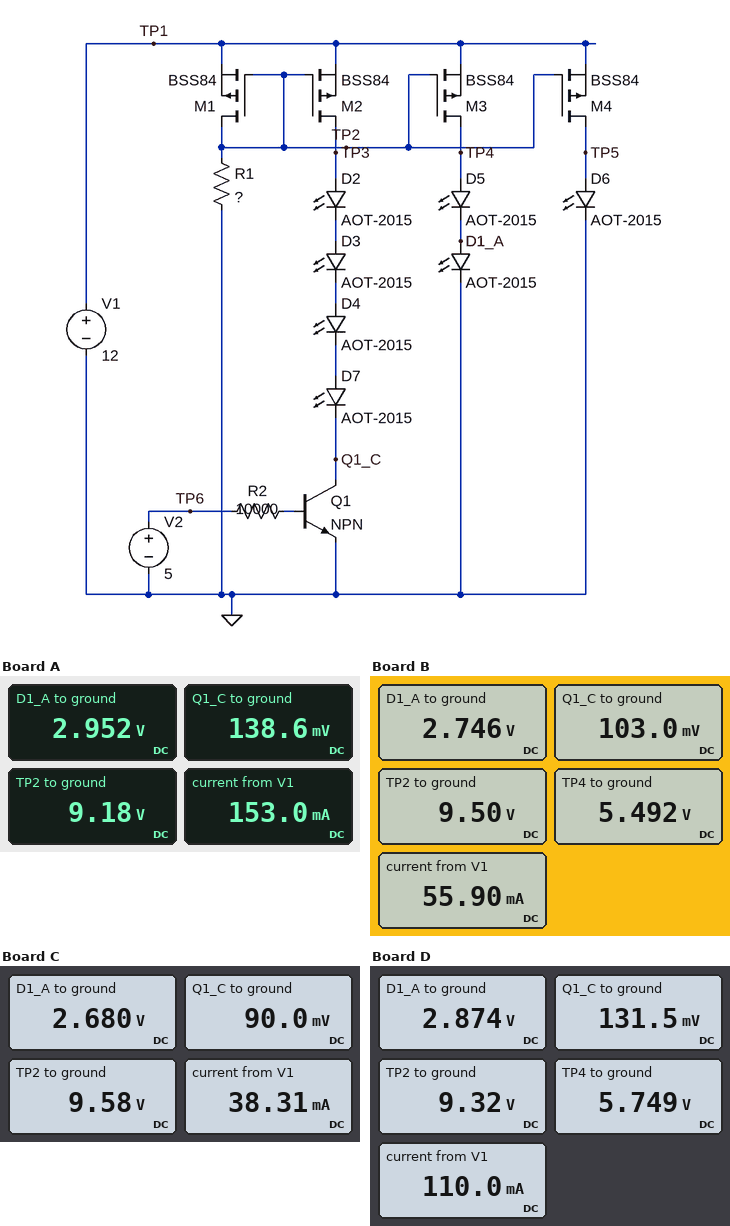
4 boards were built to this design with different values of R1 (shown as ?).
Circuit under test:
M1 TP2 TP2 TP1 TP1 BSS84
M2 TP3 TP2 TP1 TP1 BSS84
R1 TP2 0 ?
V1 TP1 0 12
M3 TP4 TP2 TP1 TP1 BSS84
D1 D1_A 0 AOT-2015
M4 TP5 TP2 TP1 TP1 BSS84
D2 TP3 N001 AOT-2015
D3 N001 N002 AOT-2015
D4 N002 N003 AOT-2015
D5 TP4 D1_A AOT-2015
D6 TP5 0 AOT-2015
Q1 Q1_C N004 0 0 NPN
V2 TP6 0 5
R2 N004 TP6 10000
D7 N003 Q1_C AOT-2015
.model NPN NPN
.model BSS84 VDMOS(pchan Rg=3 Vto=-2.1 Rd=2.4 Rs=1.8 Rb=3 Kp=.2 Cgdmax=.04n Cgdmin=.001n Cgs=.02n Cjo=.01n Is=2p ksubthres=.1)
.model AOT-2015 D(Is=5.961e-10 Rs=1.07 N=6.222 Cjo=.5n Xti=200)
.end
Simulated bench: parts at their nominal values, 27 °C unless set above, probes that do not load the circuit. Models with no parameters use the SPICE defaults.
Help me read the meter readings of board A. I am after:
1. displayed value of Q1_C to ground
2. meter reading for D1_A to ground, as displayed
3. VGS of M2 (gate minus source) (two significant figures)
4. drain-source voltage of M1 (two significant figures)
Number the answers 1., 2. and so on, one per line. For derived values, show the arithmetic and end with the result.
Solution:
1. 138.6 mV
2. 2.952 V
3. 9.18 V - 12 V = -2.8 V
4. 9.18 V - 12 V = -2.8 V
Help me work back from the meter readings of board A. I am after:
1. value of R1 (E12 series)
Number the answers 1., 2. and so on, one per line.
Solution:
1. 220 Ω
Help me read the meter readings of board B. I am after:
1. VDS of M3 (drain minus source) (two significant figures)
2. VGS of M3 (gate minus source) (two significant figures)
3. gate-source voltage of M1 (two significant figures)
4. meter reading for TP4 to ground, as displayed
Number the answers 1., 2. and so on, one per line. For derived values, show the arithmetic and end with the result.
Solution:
1. 5.492 V - 12 V = -6.5 V
2. 9.5 V - 12 V = -2.5 V
3. 9.5 V - 12 V = -2.5 V
4. 5.492 V
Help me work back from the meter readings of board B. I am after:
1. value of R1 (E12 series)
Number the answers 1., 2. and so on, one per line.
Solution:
1. 680 Ω
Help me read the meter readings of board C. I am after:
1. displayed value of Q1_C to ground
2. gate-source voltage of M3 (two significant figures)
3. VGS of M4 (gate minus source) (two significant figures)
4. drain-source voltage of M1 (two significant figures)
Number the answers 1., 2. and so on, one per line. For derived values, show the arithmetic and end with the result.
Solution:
1. 90.0 mV
2. 9.58 V - 12 V = -2.4 V
3. 9.58 V - 12 V = -2.4 V
4. 9.58 V - 12 V = -2.4 V
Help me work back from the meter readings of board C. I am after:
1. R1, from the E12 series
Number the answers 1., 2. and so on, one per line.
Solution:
1. 1 kΩ
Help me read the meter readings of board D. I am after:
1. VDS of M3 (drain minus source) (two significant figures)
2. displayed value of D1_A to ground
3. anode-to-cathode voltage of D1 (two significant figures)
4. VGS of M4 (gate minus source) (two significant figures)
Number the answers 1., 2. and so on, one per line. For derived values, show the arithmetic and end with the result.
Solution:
1. 5.749 V - 12 V = -6.3 V
2. 2.874 V
3. 2.874 V = 2.9 V
4. 9.32 V - 12 V = -2.7 V
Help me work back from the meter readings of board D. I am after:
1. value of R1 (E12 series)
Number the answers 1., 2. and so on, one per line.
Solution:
1. 330 Ω
